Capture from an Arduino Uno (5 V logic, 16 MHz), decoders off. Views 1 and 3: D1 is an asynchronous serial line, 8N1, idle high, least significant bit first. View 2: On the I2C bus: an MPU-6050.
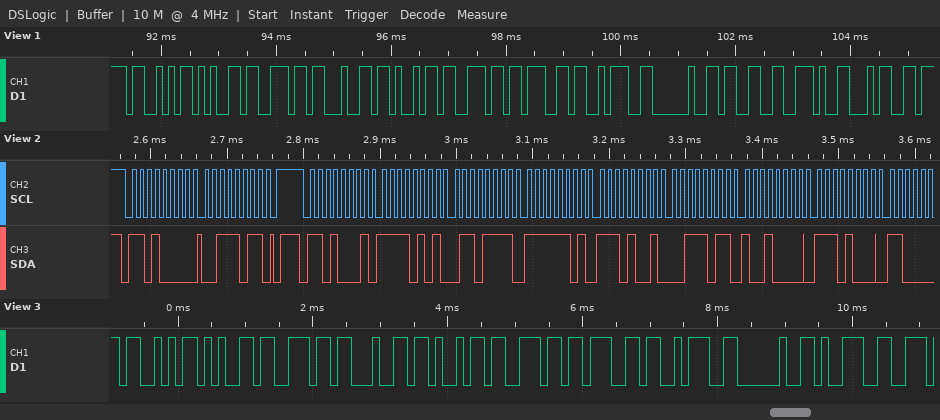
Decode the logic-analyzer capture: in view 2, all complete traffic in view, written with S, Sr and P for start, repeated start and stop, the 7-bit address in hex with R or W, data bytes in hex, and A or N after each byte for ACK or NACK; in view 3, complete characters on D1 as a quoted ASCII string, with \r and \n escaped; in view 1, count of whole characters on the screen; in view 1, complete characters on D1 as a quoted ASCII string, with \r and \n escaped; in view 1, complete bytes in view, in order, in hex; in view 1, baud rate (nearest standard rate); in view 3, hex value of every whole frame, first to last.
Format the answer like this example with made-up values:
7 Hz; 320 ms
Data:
S 68W A 3B A P S 68R A F5 A 6F A FD A E9 A 3B A 90 A E8 A; "Sending: 9"; 12; "Sending: 3.4"; 53 65 6E 64 69 6E 67 3A 20 33 2E 34; 9600 baud; 0x53 0x65 0x6E 0x64 0x69 0x6E 0x67 0x3A 0x20 0x39
